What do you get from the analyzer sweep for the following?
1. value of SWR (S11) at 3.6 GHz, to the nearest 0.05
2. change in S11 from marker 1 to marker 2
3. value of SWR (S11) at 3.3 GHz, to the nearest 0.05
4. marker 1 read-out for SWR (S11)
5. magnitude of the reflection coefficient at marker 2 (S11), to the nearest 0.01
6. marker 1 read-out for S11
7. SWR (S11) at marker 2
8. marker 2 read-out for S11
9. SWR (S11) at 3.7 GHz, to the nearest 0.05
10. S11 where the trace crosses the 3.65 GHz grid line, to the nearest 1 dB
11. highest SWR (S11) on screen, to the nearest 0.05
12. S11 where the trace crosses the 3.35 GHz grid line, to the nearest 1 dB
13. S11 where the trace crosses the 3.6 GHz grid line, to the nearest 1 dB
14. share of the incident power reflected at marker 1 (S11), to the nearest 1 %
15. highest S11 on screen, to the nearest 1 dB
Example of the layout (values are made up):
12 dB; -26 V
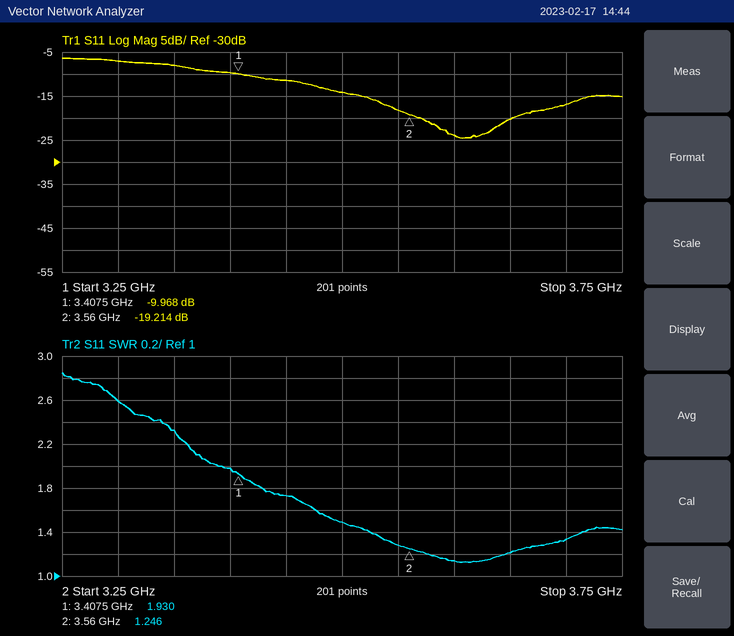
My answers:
1.15; -9.246 dB; 2.60; 1.930; 0.11; -9.968 dB; 1.246; -19.214 dB; 1.35; -20 dB; 2.85; -8 dB; -24 dB; 10 %; -6 dB
